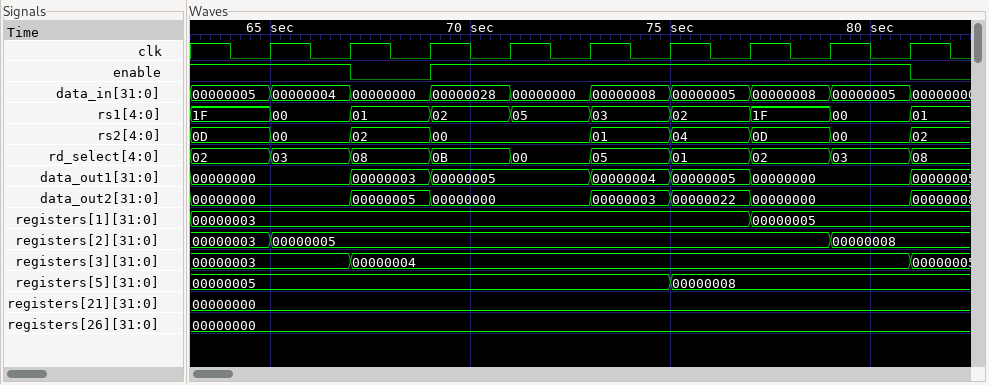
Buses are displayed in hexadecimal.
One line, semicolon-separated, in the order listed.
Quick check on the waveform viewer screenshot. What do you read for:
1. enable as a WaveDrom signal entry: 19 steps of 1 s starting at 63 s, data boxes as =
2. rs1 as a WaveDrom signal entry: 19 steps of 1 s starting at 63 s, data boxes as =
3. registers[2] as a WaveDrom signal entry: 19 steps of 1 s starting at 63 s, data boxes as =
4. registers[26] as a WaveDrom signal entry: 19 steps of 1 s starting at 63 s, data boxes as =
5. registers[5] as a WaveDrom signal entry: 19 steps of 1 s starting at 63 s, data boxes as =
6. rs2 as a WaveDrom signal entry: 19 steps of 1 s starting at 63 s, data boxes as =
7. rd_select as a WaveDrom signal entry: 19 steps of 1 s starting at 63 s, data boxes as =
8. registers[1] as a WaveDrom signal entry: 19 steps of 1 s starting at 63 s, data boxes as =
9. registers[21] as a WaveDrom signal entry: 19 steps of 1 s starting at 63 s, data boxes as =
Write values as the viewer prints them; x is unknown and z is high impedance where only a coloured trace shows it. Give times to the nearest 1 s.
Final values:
{name: 'enable', wave: '1...0.1...........0'}; {name: 'rs1', wave: '=.=.=.=.=.=.=.=.=.=', data: '1F 00 01 02 05 03 02 1F 00 01'}; {name: 'registers[2]', wave: '=.=.............=..', data: '00000003 00000005 00000008'}; {name: 'registers[26]', wave: '=..................', data: '00000000'}; {name: 'registers[5]', wave: '=...........=......', data: '00000005 00000008'}; {name: 'rs2', wave: '=.=.=.=...=.=.=.=.=', data: '0D 00 02 00 01 04 0D 00 02'}; {name: 'rd_select', wave: '=.=.=.=.=.=.=.=.=.=', data: '02 03 08 0B 00 05 01 02 03 08'}; {name: 'registers[1]', wave: '=.............=....', data: '00000003 00000005'}; {name: 'registers[21]', wave: '=..................', data: '00000000'}
